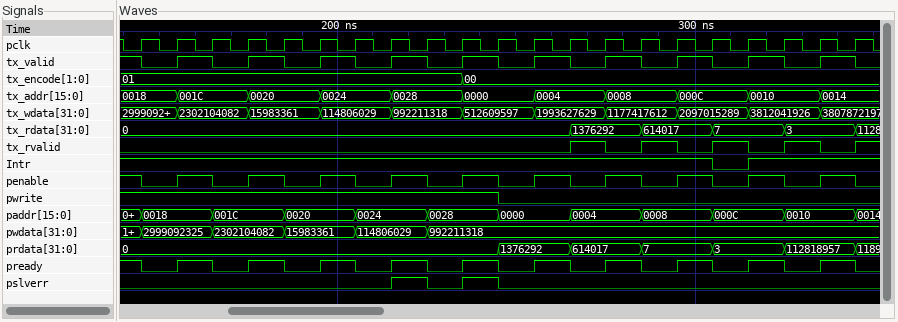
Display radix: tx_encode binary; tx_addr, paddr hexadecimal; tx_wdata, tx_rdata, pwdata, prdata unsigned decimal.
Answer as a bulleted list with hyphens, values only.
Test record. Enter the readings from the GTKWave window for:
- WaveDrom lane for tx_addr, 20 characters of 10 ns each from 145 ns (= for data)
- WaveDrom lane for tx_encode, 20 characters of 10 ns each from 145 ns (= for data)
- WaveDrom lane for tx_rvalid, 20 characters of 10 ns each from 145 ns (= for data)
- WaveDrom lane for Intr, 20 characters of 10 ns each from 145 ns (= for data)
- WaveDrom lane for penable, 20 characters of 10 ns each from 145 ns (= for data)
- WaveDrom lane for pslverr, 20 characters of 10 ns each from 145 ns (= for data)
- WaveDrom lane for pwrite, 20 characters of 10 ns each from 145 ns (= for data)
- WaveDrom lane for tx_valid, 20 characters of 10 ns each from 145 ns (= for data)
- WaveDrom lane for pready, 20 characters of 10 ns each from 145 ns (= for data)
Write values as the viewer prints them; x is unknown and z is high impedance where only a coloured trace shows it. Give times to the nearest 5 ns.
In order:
- {name: 'tx_addr', wave: '==.=.=.=.=.=.=.=.=.=', data: '0018 001C 0020 0024 0028 0000 0004 0008 000C 0010 0014'}
- {name: 'tx_encode', wave: '=........=..........', data: '01 00'}
- {name: 'tx_rvalid', wave: '0...........10101010'}
- {name: 'Intr', wave: '1...............01..'}
- {name: 'penable', wave: '01010101010101010101'}
- {name: 'pslverr', wave: '0......1010.........'}
- {name: 'pwrite', wave: '1.........0.........'}
- {name: 'tx_valid', wave: '01010101010101010101'}
- {name: 'pready', wave: '01010101010101010101'}
